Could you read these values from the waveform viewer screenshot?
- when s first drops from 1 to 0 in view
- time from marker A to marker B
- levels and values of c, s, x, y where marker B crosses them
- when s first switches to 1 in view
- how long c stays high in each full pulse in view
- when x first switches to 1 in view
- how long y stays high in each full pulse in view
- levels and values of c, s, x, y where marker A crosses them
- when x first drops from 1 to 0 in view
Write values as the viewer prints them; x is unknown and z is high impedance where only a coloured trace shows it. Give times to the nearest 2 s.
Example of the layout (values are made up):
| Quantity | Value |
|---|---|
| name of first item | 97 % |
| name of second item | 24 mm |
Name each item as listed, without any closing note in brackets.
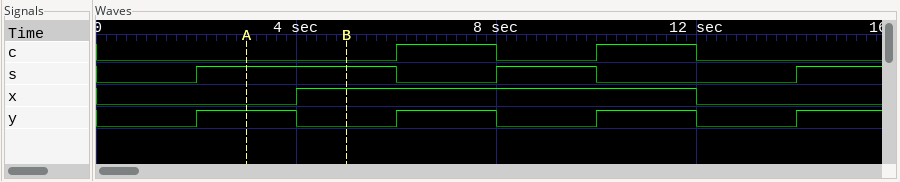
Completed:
| Quantity | Value |
|---|---|
| when s first drops from 1 to 0 in view | 6 s |
| time from marker A to marker B | 2 s |
| levels and values of c, s, x, y where marker B crosses them | c=0, s=1, x=1, y=0 |
| when s first switches to 1 in view | 2 s |
| how long c stays high in each full pulse in view | 2 s, 2 s |
| when x first switches to 1 in view | 4 s |
| how long y stays high in each full pulse in view | 2 s, 2 s, 2 s |
| levels and values of c, s, x, y where marker A crosses them | c=0, s=1, x=0, y=1 |
| when x first drops from 1 to 0 in view | 12 s |
